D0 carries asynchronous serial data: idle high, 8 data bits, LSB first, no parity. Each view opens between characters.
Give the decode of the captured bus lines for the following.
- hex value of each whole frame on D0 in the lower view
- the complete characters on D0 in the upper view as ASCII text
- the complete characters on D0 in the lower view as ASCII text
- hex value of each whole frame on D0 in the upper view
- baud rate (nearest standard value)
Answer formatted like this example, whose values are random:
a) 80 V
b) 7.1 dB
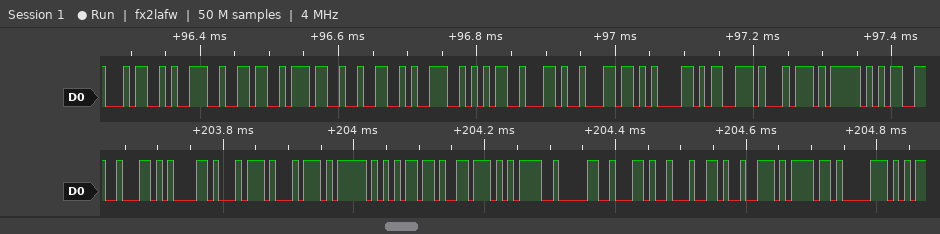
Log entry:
a) 62, 61, 74, 74, 5F, 6D, 76, 3D, 30, 2C, 64, 72, 6F, 70
b) "4967295,last_"
c) "batt_mv=0,drop"
d) 34, 39, 36, 37, 32, 39, 35, 2C, 6C, 61, 73, 74, 5F
e) 115200 baud
